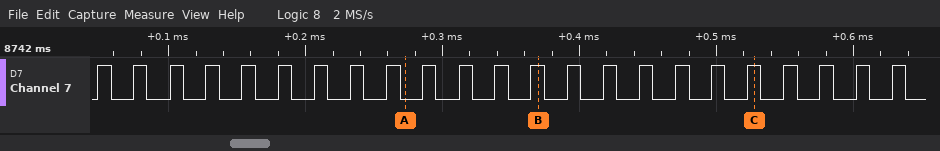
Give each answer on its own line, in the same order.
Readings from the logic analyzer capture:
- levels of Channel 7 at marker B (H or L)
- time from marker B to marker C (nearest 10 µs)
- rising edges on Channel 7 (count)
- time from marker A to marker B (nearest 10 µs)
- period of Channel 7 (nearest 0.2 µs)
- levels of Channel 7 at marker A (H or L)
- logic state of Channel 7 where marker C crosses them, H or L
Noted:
Channel 7=H
160 µs
23
100 µs
26.4 µs
Channel 7=L
Channel 7=H
